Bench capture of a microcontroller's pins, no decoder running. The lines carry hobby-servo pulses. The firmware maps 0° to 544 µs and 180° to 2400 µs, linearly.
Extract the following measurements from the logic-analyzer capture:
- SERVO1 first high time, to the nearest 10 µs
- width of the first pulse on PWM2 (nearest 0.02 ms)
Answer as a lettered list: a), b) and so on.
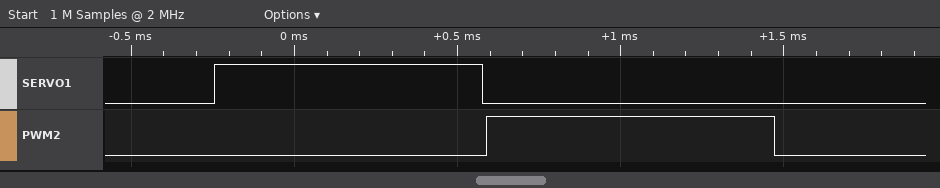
a) 820 µs
b) 0.88 ms
